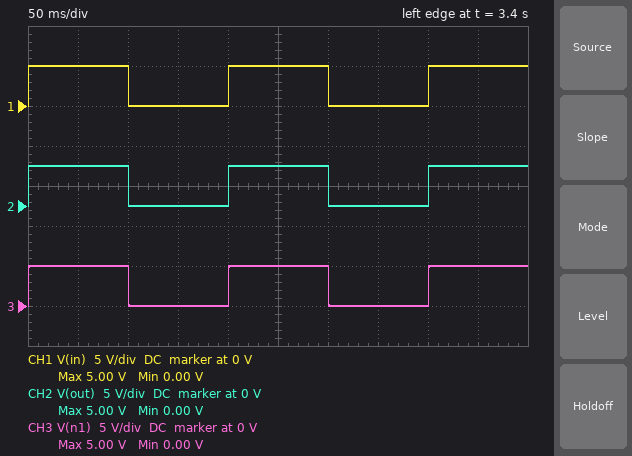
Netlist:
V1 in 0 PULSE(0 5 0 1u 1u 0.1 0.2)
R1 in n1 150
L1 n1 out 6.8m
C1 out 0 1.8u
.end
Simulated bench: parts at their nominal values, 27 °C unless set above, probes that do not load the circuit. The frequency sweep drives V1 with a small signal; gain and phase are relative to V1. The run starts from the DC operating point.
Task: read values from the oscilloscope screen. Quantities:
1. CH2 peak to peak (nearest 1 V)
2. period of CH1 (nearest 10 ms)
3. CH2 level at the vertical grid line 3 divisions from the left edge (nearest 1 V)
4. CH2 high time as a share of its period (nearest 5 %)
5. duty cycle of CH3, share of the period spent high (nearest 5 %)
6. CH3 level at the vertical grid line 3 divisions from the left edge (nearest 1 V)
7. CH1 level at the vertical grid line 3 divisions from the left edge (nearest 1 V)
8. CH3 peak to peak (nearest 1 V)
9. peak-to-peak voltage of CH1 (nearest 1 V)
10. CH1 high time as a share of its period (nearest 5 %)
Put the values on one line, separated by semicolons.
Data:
5 V; 200 ms; 0 V; 50 %; 50 %; 0 V; 0 V; 5 V; 5 V; 50 %
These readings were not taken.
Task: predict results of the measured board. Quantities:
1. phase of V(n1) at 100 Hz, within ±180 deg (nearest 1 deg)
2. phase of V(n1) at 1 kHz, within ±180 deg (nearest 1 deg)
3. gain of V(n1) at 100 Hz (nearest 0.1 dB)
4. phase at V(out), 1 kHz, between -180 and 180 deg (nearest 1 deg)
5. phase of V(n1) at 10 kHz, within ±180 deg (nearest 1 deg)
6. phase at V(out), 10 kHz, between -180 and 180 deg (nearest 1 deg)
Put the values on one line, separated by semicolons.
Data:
-10 deg; -73 deg; -0.1 dB; -73 deg; 20 deg; -160 deg
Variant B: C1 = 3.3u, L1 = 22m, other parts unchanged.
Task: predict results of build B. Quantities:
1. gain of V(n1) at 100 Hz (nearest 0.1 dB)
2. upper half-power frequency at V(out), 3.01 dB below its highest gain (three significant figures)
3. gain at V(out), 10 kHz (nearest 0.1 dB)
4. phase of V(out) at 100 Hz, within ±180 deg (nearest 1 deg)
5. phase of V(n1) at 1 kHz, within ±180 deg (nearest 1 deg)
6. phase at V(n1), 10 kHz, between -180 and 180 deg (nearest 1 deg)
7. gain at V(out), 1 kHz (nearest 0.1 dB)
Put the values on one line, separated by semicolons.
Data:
-0.4 dB; 428 Hz; -49.2 dB; -18 deg; 59 deg; 6 deg; -11.2 dB
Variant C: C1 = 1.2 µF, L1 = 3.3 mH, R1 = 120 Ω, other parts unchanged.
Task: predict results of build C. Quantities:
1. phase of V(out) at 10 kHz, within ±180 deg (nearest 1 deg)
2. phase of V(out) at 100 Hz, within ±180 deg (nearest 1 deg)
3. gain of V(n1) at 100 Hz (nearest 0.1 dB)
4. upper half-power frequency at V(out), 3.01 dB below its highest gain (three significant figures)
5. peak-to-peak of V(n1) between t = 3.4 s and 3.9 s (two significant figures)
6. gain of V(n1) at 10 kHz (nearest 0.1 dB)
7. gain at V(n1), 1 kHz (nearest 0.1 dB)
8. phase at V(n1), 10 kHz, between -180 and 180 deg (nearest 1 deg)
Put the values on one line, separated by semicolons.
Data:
-148 deg; -5 deg; 0 dB; 1.35 kHz; 5.0 V; -1.4 dB; -3.3 dB; 32 deg
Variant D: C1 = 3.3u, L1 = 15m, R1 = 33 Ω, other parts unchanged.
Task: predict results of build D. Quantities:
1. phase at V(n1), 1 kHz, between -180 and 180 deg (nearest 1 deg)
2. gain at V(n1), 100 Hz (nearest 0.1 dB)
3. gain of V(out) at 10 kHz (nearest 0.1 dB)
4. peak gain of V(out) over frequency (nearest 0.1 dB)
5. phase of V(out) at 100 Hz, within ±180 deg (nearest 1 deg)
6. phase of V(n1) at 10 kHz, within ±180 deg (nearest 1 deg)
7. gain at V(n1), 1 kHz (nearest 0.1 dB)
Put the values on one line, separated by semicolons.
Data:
36 deg; 0 dB; -45.8 dB; 6.5 dB; -4 deg; 2 deg; -1.8 dB
